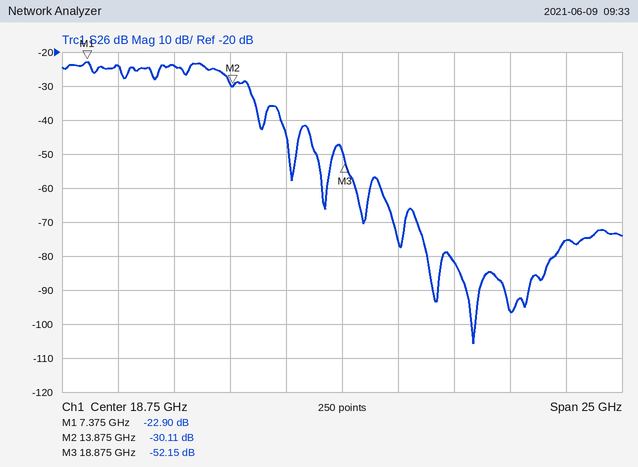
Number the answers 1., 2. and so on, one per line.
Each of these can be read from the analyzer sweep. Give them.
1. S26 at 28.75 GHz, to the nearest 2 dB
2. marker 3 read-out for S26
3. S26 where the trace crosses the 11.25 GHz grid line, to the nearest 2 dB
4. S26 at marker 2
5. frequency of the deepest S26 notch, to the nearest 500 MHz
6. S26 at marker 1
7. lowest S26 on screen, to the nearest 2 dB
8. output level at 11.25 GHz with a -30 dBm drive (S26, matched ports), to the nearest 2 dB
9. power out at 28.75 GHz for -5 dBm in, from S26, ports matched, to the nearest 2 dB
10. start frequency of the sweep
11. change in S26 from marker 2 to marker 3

1. -76 dB
2. -52.15 dB
3. -24 dB
4. -30.11 dB
5. 24.5 GHz
6. -22.90 dB
7. -106 dB
8. -54 dBm
9. -80 dBm
10. 6.25 GHz
11. -22.04 dB
